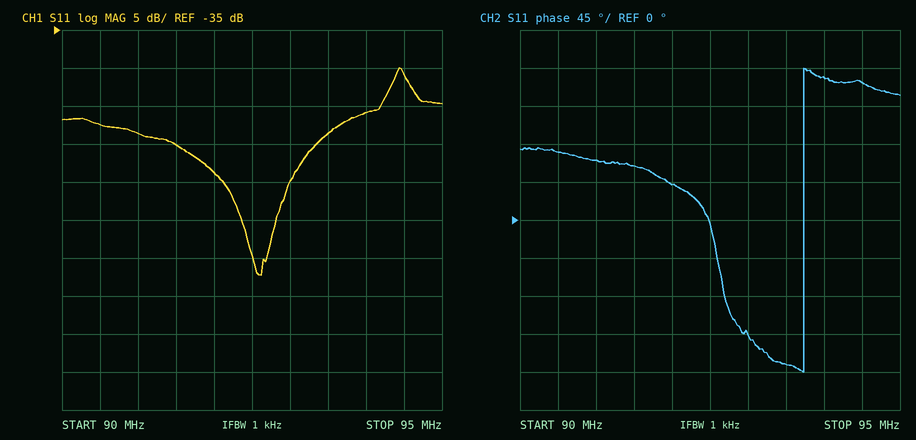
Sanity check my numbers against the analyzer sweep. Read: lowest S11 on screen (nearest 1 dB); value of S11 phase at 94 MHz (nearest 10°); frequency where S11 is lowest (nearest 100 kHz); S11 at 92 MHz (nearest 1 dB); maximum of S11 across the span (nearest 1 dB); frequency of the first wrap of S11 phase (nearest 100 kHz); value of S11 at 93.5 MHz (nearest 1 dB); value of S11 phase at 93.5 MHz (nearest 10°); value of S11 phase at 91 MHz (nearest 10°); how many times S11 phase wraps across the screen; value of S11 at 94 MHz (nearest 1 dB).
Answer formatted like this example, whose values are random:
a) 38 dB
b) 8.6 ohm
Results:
a) -67 dB
b) 170°
c) 92.6 MHz
d) -54 dB
e) -40 dB
f) 93.7 MHz
g) -49 dB
h) -170°
i) 70°
j) 1
k) -46 dB
